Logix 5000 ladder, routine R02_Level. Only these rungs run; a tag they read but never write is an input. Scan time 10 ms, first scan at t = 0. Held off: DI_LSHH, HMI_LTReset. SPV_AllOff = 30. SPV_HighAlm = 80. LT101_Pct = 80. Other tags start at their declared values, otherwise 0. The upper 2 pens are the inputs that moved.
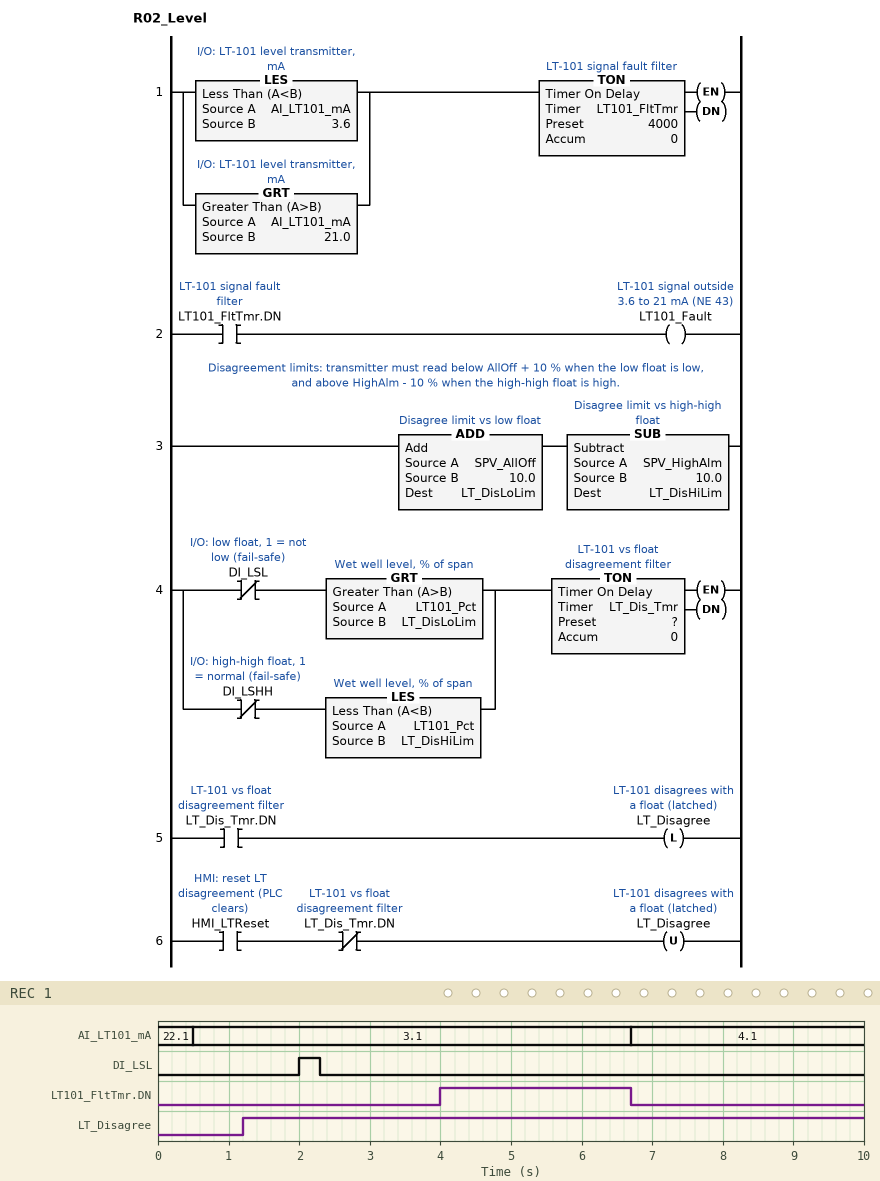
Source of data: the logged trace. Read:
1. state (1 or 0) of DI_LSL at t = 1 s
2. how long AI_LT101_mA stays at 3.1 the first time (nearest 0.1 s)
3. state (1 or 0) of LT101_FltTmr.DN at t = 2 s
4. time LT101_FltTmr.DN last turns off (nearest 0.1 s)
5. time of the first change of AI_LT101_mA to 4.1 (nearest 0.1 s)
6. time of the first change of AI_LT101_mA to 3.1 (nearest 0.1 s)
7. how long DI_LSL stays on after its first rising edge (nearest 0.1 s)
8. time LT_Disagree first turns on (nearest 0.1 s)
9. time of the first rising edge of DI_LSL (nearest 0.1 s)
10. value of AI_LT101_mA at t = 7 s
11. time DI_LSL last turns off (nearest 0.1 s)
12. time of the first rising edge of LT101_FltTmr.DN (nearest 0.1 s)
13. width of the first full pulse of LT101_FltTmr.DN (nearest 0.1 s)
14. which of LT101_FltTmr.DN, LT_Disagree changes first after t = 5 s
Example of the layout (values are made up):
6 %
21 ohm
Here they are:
0
6.2 s
0
6.7 s
6.7 s
0.5 s
0.3 s
1.2 s
2.0 s
4.1
2.3 s
4.0 s
2.7 s
LT101_FltTmr.DN
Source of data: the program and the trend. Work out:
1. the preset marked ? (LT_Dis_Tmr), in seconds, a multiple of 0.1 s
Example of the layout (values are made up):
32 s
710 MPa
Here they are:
1.2 s
